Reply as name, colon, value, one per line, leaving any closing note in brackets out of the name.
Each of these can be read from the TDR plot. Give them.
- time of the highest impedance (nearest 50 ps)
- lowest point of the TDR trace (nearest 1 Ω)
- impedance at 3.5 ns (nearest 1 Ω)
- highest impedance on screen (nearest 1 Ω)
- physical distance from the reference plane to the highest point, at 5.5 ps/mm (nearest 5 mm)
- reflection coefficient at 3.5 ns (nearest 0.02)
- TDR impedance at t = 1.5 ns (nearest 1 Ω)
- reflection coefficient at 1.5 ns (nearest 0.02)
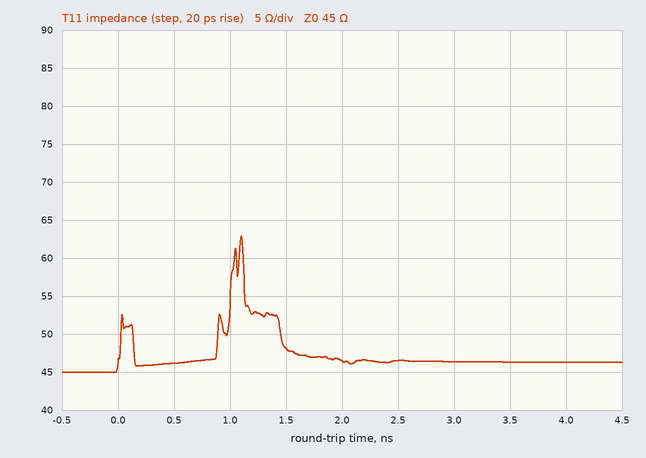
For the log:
time of the highest impedance: 1.10 ns
lowest point of the TDR trace: 45 Ω
impedance at 3.5 ns: 46 Ω
highest impedance on screen: 63 Ω
physical distance from the reference plane to the highest point, at 5.5 ps/mm: 100 mm
reflection coefficient at 3.5 ns: +0.02
TDR impedance at t = 1.5 ns: 48 Ω
reflection coefficient at 1.5 ns: +0.04
